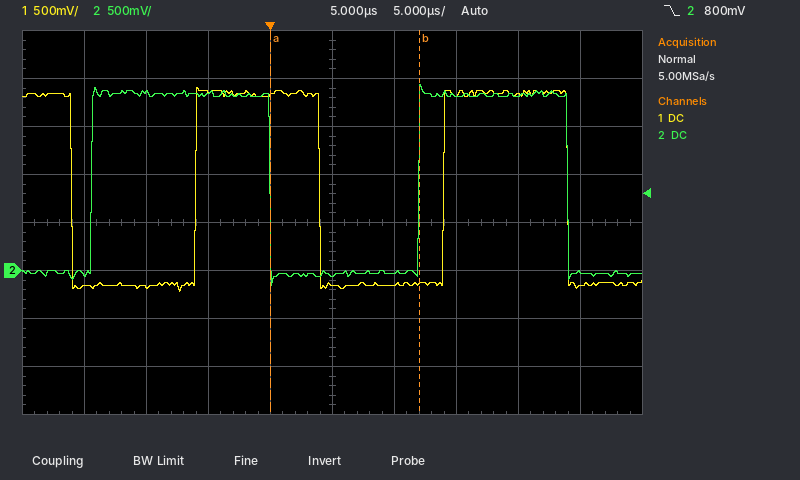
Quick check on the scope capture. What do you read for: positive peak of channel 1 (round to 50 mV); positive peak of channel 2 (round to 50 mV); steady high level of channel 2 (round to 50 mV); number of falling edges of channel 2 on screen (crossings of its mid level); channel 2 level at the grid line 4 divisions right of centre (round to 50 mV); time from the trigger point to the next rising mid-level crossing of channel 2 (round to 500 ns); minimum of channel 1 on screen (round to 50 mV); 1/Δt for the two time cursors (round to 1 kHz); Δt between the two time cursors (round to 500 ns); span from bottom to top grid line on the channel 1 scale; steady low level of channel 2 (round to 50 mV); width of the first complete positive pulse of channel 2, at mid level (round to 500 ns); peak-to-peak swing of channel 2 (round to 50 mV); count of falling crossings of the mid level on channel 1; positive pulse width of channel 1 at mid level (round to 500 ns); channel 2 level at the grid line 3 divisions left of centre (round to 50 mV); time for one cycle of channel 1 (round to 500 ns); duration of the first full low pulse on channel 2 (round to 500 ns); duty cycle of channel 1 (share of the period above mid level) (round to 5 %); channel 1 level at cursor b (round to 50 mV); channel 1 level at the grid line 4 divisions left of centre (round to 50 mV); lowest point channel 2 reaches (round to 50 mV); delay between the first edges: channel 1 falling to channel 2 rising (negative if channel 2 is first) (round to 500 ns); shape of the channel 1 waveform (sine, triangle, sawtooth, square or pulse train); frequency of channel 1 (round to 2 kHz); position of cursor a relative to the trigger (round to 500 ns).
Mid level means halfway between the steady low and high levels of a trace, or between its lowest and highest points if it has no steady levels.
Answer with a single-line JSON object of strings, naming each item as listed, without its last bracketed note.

{"positive peak of channel 1": "1.90 V", "positive peak of channel 2": "1.95 V", "steady high level of channel 2": "1.85 V", "number of falling edges of channel 2 on screen": "2", "channel 2 level at the grid line 4 divisions right of centre": "0 mV", "time from the trigger point to the next rising mid-level crossing of channel 2": "12.0 µs", "minimum of channel 1 on screen": "-200 mV", "1/Δt for the two time cursors": "83 kHz", "Δt between the two time cursors": "12.0 µs", "span from bottom to top grid line on the channel 1 scale": "4 V", "steady low level of channel 2": "-50 mV", "width of the first complete positive pulse of channel 2, at mid level": "14.5 µs", "peak-to-peak swing of channel 2": "2.10 V", "count of falling crossings of the mid level on channel 1": "3", "positive pulse width of channel 1 at mid level": "10.0 µs", "channel 2 level at the grid line 3 divisions left of centre": "1.85 V", "time for one cycle of channel 1": "20.0 µs", "duration of the first full low pulse on channel 2": "12.0 µs", "duty cycle of channel 1 (share of the period above mid level)": "50 %", "channel 1 level at cursor b": "-150 mV", "channel 1 level at the grid line 4 divisions left of centre": "-150 mV", "lowest point channel 2 reaches": "-150 mV", "delay between the first edges: channel 1 falling to channel 2 rising (negative if channel 2 is first)": "+1.5 µs", "shape of the channel 1 waveform": "square", "frequency of channel 1": "50 kHz", "position of cursor a relative to the trigger": "0.0 µs"}
